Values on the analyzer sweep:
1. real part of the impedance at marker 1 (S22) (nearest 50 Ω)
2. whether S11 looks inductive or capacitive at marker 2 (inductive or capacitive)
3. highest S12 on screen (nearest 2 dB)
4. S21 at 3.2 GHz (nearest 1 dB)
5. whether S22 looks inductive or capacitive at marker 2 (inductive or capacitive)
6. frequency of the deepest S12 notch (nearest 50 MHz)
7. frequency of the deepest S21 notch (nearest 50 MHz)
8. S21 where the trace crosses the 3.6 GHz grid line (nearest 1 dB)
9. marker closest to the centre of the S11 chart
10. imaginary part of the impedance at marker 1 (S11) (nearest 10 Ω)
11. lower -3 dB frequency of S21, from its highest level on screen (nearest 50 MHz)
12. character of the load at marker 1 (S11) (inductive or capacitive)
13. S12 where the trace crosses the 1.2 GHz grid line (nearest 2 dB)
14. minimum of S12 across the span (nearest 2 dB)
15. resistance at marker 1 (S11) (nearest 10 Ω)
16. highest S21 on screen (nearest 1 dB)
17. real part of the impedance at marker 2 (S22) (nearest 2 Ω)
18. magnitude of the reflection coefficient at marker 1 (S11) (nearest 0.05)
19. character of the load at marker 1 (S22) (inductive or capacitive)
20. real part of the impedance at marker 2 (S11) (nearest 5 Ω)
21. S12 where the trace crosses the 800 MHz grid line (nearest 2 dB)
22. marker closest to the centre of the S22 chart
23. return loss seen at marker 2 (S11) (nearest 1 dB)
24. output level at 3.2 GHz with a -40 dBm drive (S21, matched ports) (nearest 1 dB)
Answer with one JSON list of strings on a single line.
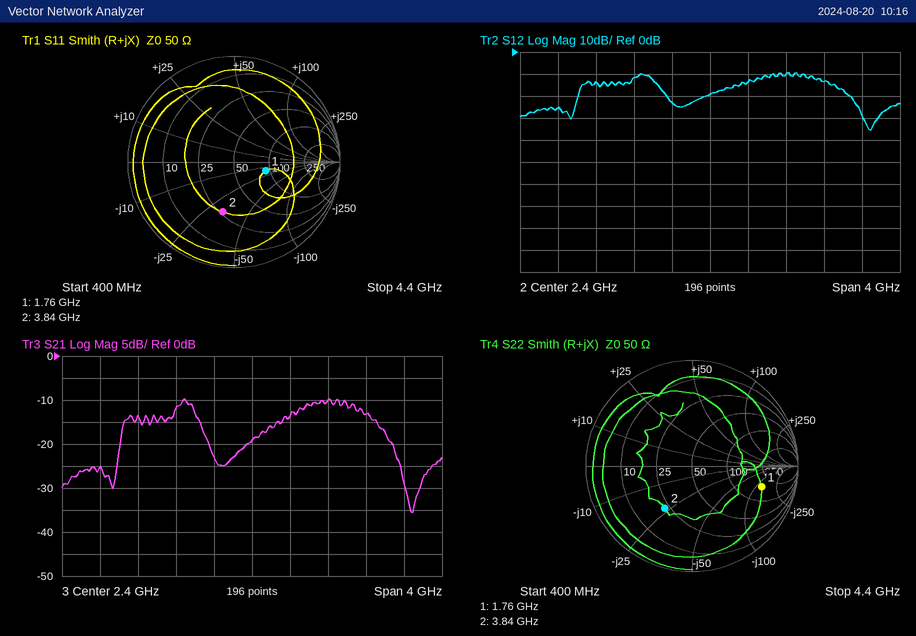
["150 Ω", "capacitive", "-10 dB", "-10 dB", "capacitive", "4.10 GHz", "4.10 GHz", "-13 dB", "marker 1", "-20 Ω", "1.60 GHz", "capacitive", "-14 dB", "-36 dB", "90 Ω", "-10 dB", "22 Ω", "0.30", "capacitive", "25 Ω", "-26 dB", "marker 2", "6 dB", "-50 dBm"]
